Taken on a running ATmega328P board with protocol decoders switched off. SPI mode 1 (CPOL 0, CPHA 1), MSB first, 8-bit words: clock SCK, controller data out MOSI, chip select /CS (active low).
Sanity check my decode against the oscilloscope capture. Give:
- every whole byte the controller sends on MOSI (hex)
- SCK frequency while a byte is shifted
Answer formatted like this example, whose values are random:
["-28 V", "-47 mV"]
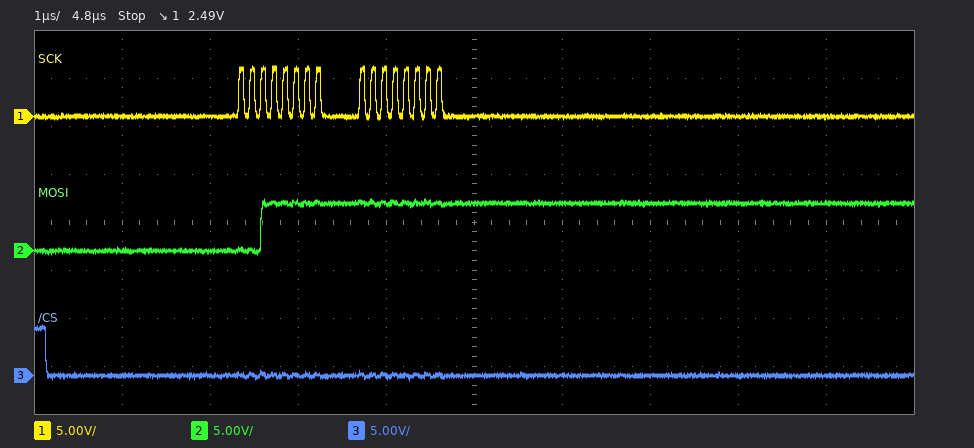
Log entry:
["3F FF", "8 MHz"]
